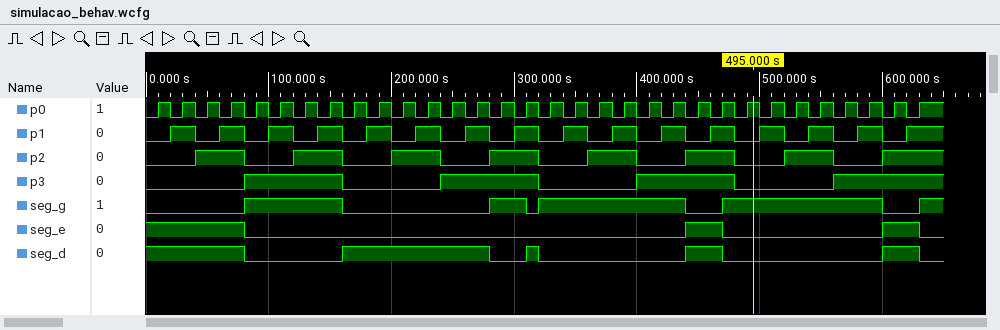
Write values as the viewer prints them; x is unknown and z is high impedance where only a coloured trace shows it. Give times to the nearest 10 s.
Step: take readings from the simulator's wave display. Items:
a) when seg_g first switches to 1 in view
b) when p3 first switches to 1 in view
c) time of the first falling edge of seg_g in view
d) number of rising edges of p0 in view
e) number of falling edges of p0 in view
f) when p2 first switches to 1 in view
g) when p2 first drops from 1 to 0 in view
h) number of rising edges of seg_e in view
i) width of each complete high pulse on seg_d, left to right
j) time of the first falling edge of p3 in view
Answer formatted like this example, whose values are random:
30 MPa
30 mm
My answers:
80 s
80 s
160 s
32
31
40 s
80 s
2
120 s, 10 s, 30 s, 30 s
160 s
